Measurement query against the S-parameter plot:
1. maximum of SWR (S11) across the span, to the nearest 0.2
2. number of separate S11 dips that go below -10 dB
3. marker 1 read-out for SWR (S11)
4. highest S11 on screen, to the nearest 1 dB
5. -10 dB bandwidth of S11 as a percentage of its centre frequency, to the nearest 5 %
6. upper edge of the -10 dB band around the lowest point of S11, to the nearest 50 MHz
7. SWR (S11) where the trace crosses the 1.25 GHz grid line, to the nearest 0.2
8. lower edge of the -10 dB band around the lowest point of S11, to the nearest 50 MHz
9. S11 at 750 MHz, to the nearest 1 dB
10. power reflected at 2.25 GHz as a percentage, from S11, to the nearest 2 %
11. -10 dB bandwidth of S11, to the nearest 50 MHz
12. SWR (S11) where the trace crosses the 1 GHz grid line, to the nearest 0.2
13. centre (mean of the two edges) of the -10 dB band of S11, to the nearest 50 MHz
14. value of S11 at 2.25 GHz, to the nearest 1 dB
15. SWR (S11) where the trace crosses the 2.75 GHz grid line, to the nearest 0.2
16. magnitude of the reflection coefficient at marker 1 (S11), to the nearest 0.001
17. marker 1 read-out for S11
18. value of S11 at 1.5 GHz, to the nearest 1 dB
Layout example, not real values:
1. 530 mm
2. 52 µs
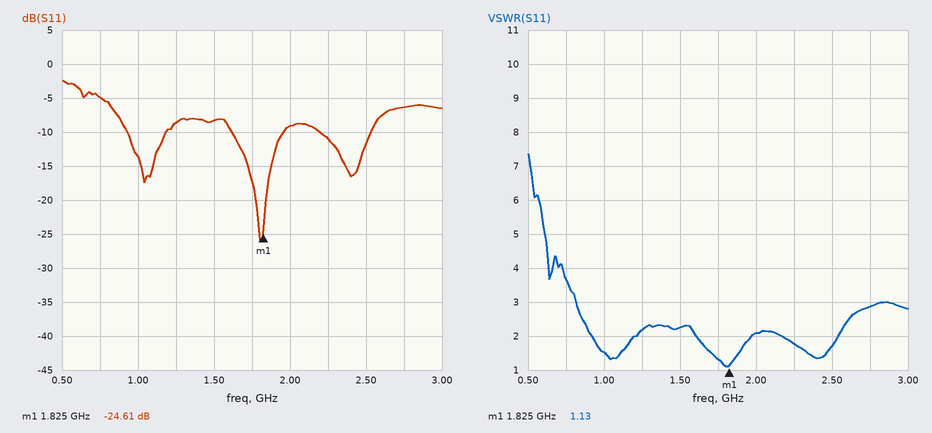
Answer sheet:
1. 7.4
2. 3
3. 1.13
4. -2 dB
5. 20 %
6. 1.95 GHz
7. 2.2
8. 1.60 GHz
9. -5 dB
10. 8 %
11. 350 MHz
12. 1.6
13. 1.80 GHz
14. -11 dB
15. 2.8
16. 0.059
17. -24.61 dB
18. -8 dB
